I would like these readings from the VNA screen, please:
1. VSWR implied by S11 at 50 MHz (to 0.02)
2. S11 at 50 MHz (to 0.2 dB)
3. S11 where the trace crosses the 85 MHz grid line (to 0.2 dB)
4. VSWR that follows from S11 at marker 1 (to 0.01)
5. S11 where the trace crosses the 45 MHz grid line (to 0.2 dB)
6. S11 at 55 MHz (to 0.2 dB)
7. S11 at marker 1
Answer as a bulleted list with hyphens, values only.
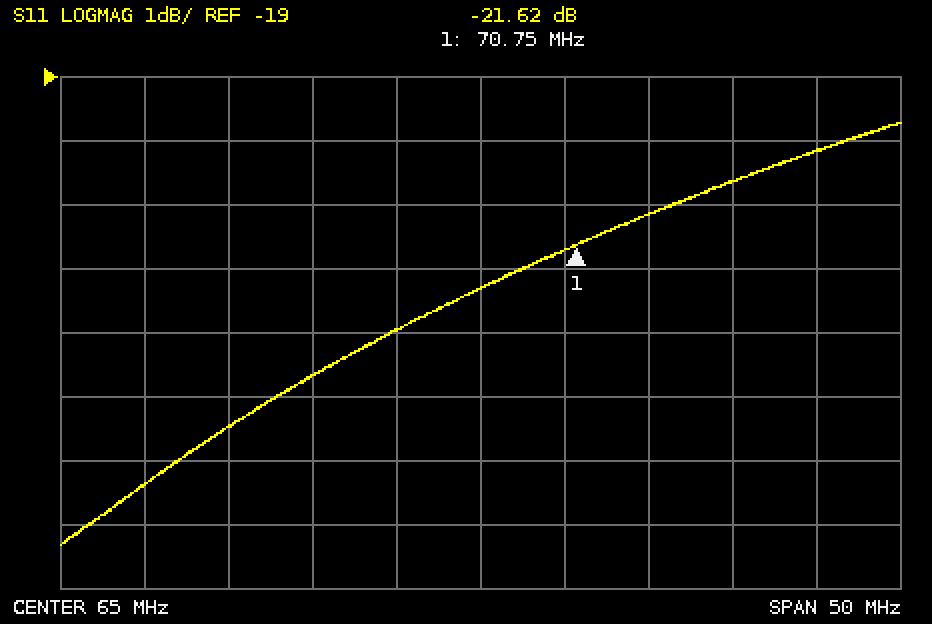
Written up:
- 1.12
- -24.4 dB
- -20.2 dB
- 1.18
- -25.4 dB
- -23.6 dB
- -21.62 dB
